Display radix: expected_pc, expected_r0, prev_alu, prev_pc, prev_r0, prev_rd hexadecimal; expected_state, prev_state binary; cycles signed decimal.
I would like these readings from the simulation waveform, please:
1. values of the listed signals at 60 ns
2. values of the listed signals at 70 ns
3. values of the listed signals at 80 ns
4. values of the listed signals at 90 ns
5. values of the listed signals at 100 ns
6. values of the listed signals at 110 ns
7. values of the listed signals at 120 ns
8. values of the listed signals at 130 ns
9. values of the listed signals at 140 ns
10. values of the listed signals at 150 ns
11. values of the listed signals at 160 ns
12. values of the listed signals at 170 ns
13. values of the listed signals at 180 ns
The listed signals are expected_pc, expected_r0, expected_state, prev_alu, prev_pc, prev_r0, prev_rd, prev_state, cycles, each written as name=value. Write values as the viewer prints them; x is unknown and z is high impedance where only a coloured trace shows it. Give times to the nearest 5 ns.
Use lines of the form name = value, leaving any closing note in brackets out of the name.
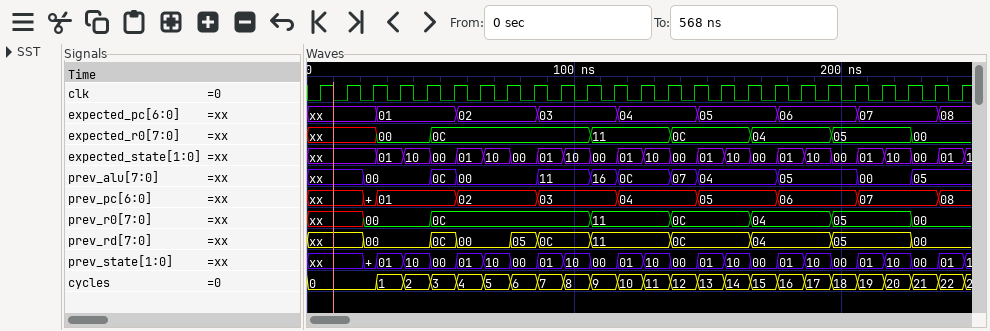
values of the listed signals at 60 ns = expected_pc=02, expected_r0=0C, expected_state=01, prev_alu=00, prev_pc=02, prev_r0=0C, prev_rd=00, prev_state=01, cycles=4
values of the listed signals at 70 ns = expected_pc=02, expected_r0=0C, expected_state=10, prev_alu=00, prev_pc=02, prev_r0=0C, prev_rd=00, prev_state=10, cycles=5
values of the listed signals at 80 ns = expected_pc=02, expected_r0=0C, expected_state=00, prev_alu=00, prev_pc=02, prev_r0=0C, prev_rd=05, prev_state=00, cycles=6
values of the listed signals at 90 ns = expected_pc=03, expected_r0=0C, expected_state=01, prev_alu=11, prev_pc=03, prev_r0=0C, prev_rd=0C, prev_state=01, cycles=7
values of the listed signals at 100 ns = expected_pc=03, expected_r0=0C, expected_state=10, prev_alu=11, prev_pc=03, prev_r0=0C, prev_rd=0C, prev_state=10, cycles=8
values of the listed signals at 110 ns = expected_pc=03, expected_r0=11, expected_state=00, prev_alu=16, prev_pc=03, prev_r0=11, prev_rd=11, prev_state=00, cycles=9
values of the listed signals at 120 ns = expected_pc=04, expected_r0=11, expected_state=01, prev_alu=0C, prev_pc=04, prev_r0=11, prev_rd=11, prev_state=01, cycles=10
values of the listed signals at 130 ns = expected_pc=04, expected_r0=11, expected_state=10, prev_alu=0C, prev_pc=04, prev_r0=11, prev_rd=11, prev_state=10, cycles=11
values of the listed signals at 140 ns = expected_pc=04, expected_r0=0C, expected_state=00, prev_alu=07, prev_pc=04, prev_r0=0C, prev_rd=0C, prev_state=00, cycles=12
values of the listed signals at 150 ns = expected_pc=05, expected_r0=0C, expected_state=01, prev_alu=04, prev_pc=05, prev_r0=0C, prev_rd=0C, prev_state=01, cycles=13
values of the listed signals at 160 ns = expected_pc=05, expected_r0=0C, expected_state=10, prev_alu=04, prev_pc=05, prev_r0=0C, prev_rd=0C, prev_state=10, cycles=14
values of the listed signals at 170 ns = expected_pc=05, expected_r0=04, expected_state=00, prev_alu=04, prev_pc=05, prev_r0=04, prev_rd=04, prev_state=00, cycles=15
values of the listed signals at 180 ns = expected_pc=06, expected_r0=04, expected_state=01, prev_alu=05, prev_pc=06, prev_r0=04, prev_rd=04, prev_state=01, cycles=16
